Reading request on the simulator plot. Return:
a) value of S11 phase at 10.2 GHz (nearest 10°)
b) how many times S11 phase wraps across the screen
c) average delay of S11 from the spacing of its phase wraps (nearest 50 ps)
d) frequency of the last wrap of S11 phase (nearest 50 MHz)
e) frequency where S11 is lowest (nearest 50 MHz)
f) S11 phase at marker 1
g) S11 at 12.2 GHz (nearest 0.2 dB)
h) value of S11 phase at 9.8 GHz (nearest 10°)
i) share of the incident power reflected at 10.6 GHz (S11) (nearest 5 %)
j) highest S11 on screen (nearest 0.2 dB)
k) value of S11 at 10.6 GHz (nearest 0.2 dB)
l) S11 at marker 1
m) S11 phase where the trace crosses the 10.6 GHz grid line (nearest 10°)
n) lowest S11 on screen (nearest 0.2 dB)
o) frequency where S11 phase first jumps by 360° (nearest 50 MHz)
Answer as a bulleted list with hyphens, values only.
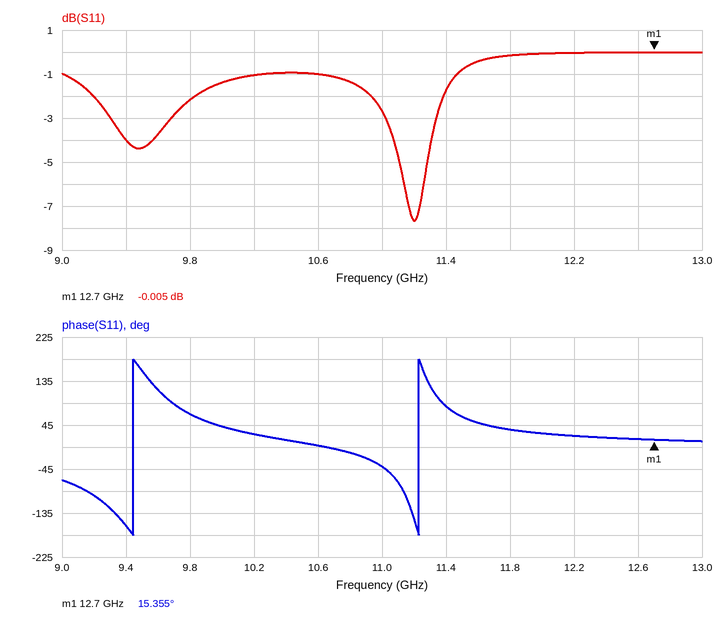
- 30°
- 2
- 550 ps
- 11.25 GHz
- 11.20 GHz
- 15.355°
- 0.0 dB
- 70°
- 80 %
- 0.0 dB
- -1.0 dB
- -0.005 dB
- 0°
- -7.6 dB
- 9.45 GHz
